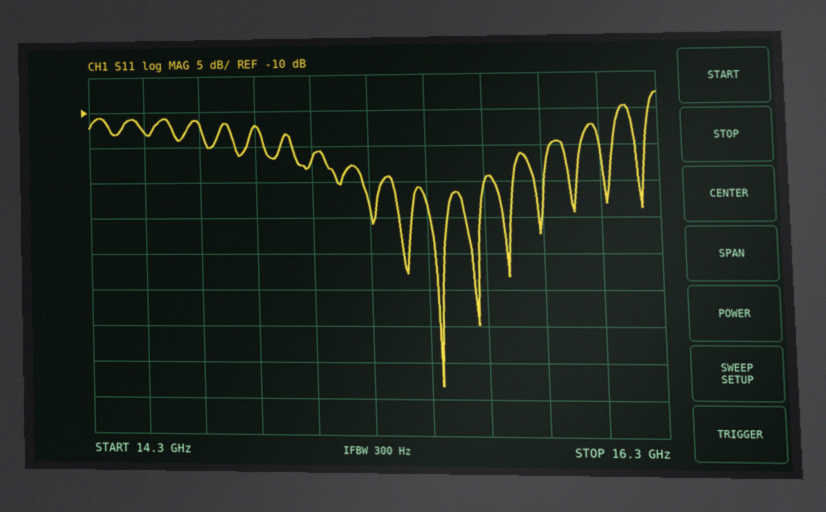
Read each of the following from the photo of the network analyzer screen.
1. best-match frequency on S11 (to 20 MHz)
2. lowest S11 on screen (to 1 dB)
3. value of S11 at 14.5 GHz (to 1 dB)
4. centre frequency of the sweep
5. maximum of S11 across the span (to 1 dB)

15.54 GHz
-48 dB
-13 dB
15.3 GHz
-8 dB
